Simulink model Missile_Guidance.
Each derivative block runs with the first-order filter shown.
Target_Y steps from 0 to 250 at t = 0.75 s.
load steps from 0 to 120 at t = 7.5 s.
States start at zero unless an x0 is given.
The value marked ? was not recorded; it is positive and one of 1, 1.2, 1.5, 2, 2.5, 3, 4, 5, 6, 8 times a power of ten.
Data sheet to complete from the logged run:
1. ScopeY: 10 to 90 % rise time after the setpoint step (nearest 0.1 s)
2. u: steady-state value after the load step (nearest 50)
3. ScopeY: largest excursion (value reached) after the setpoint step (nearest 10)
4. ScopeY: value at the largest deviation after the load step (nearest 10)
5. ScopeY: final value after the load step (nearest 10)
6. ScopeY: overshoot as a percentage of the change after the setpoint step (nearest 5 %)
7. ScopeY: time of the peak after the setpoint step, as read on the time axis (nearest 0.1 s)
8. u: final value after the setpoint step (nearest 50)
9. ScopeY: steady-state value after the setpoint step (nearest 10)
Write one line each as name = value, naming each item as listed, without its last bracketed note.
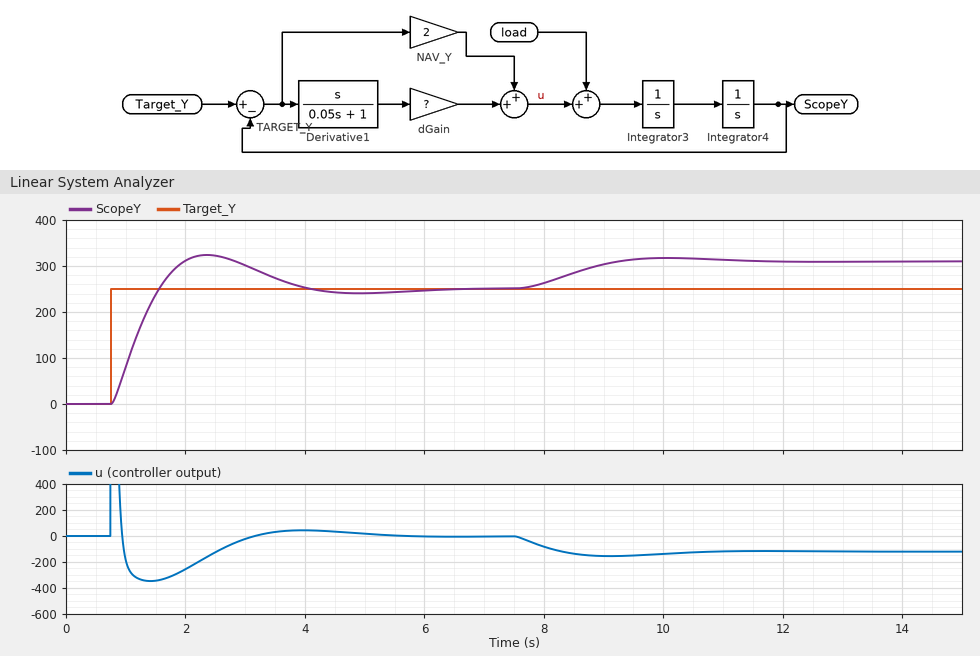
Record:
ScopeY: 10 to 90 % rise time after the setpoint step = 0.6 s
u: steady-state value after the load step = -100
ScopeY: largest excursion (value reached) after the setpoint step = 320
ScopeY: value at the largest deviation after the load step = 320
ScopeY: final value after the load step = 310
ScopeY: overshoot as a percentage of the change after the setpoint step = 30 %
ScopeY: time of the peak after the setpoint step, as read on the time axis = 2.4 s
u: final value after the setpoint step = 0
ScopeY: steady-state value after the setpoint step = 250
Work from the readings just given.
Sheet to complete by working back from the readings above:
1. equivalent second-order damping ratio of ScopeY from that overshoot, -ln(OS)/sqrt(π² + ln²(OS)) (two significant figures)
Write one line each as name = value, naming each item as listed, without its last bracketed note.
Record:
equivalent second-order damping ratio of ScopeY from that overshoot, -ln(OS)/sqrt(π² + ln²(OS)) = 0.36
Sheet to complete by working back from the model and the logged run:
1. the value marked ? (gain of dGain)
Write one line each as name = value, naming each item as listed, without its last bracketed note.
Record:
the value marked ? = 1.5
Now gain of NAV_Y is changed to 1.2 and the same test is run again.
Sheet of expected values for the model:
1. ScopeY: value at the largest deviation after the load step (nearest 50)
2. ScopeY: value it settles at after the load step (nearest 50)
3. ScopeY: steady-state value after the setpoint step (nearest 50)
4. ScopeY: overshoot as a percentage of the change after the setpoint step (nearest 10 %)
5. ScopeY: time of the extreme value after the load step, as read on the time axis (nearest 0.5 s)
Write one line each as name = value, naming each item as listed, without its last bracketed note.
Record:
ScopeY: value at the largest deviation after the load step = 350
ScopeY: value it settles at after the load step = 350
ScopeY: steady-state value after the setpoint step = 250
ScopeY: overshoot as a percentage of the change after the setpoint step = 20 %
ScopeY: time of the extreme value after the load step, as read on the time axis = 11.5 s
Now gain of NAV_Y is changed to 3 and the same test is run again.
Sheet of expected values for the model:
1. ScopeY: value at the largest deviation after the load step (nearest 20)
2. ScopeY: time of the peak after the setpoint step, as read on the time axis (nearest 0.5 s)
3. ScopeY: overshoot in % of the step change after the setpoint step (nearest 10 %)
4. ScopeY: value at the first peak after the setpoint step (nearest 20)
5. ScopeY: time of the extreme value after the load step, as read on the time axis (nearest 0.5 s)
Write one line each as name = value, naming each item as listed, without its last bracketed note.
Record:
ScopeY: value at the largest deviation after the load step = 300
ScopeY: time of the peak after the setpoint step, as read on the time axis = 2.0 s
ScopeY: overshoot in % of the step change after the setpoint step = 40 %
ScopeY: value at the first peak after the setpoint step = 340
ScopeY: time of the extreme value after the load step, as read on the time axis = 9.5 s
